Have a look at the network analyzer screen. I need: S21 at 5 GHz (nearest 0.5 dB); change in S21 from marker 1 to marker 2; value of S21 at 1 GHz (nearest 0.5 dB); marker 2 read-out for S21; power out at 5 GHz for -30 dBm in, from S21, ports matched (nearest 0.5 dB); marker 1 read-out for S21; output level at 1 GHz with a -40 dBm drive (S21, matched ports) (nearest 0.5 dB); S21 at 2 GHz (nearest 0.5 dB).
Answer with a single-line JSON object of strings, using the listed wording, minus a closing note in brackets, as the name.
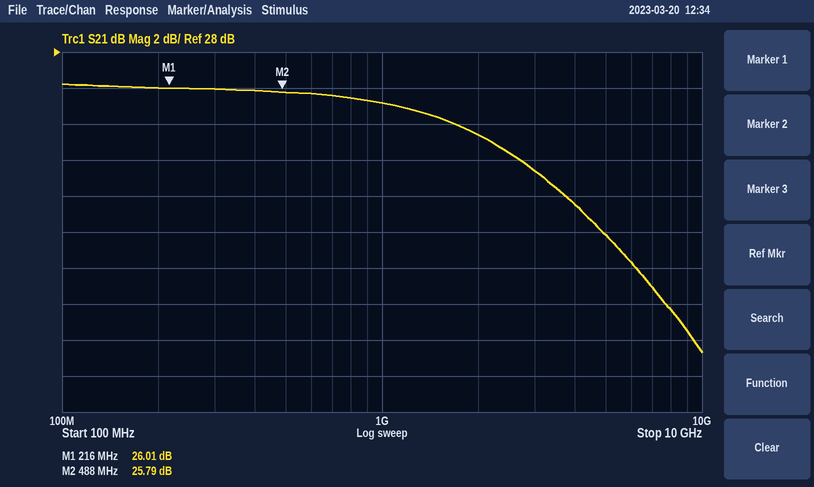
{"S21 at 5 GHz": "18.0 dB", "change in S21 from marker 1 to marker 2": "-0.22 dB", "value of S21 at 1 GHz": "25.0 dB", "marker 2 read-out for S21": "25.79 dB", "power out at 5 GHz for -30 dBm in, from S21, ports matched": "-12.0 dBm", "marker 1 read-out for S21": "26.01 dB", "output level at 1 GHz with a -40 dBm drive (S21, matched ports)": "-15.0 dBm", "S21 at 2 GHz": "23.5 dB"}
